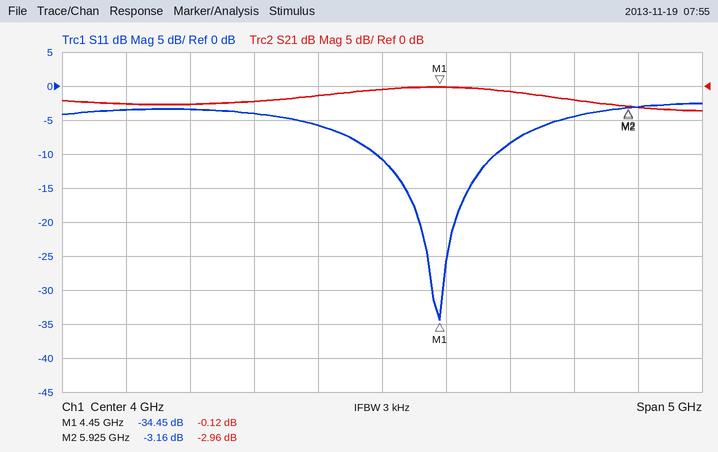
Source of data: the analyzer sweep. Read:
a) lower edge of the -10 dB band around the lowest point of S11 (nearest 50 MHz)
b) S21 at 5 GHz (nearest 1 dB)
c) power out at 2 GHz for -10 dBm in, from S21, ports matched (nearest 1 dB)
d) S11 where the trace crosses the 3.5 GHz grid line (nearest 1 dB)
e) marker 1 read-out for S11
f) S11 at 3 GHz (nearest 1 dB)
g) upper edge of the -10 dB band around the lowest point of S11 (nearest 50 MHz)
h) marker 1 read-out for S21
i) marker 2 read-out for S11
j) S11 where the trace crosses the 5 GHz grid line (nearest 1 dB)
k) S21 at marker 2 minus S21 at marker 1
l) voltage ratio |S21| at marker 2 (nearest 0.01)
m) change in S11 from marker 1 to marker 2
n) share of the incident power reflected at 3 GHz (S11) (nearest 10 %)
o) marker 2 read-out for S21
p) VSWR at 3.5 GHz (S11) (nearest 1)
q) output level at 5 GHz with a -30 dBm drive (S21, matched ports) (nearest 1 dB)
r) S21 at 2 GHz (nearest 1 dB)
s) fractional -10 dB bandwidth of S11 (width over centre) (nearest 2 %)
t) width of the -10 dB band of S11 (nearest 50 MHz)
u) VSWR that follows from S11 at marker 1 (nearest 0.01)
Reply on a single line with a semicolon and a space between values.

3.95 GHz; -1 dB; -13 dBm; -6 dB; -34.45 dB; -4 dB; 4.90 GHz; -0.12 dB; -3.16 dB; -8 dB; -2.84 dB; 0.71; 31.29 dB; 40 %; -2.96 dB; 3; -31 dBm; -3 dB; 22 %; 950 MHz; 1.04
